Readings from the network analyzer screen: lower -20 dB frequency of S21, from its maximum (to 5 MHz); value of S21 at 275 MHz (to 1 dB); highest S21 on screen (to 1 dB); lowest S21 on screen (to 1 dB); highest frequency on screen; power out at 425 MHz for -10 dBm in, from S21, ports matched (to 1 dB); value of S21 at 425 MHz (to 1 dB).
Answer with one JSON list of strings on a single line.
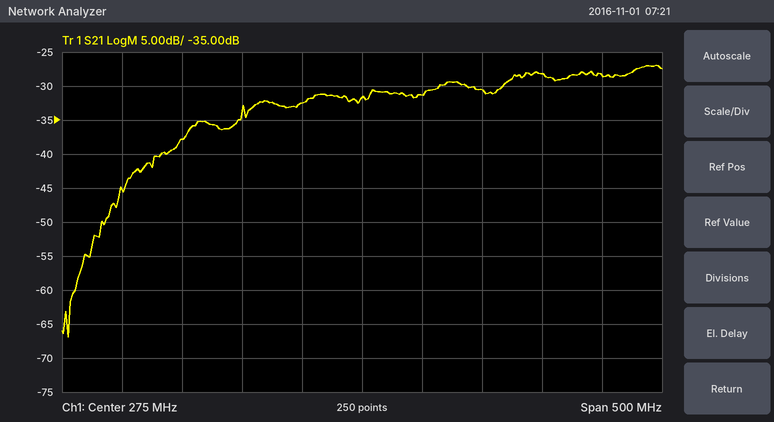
["70 MHz", "-32 dB", "-27 dB", "-67 dB", "525 MHz", "-38 dBm", "-28 dB"]
